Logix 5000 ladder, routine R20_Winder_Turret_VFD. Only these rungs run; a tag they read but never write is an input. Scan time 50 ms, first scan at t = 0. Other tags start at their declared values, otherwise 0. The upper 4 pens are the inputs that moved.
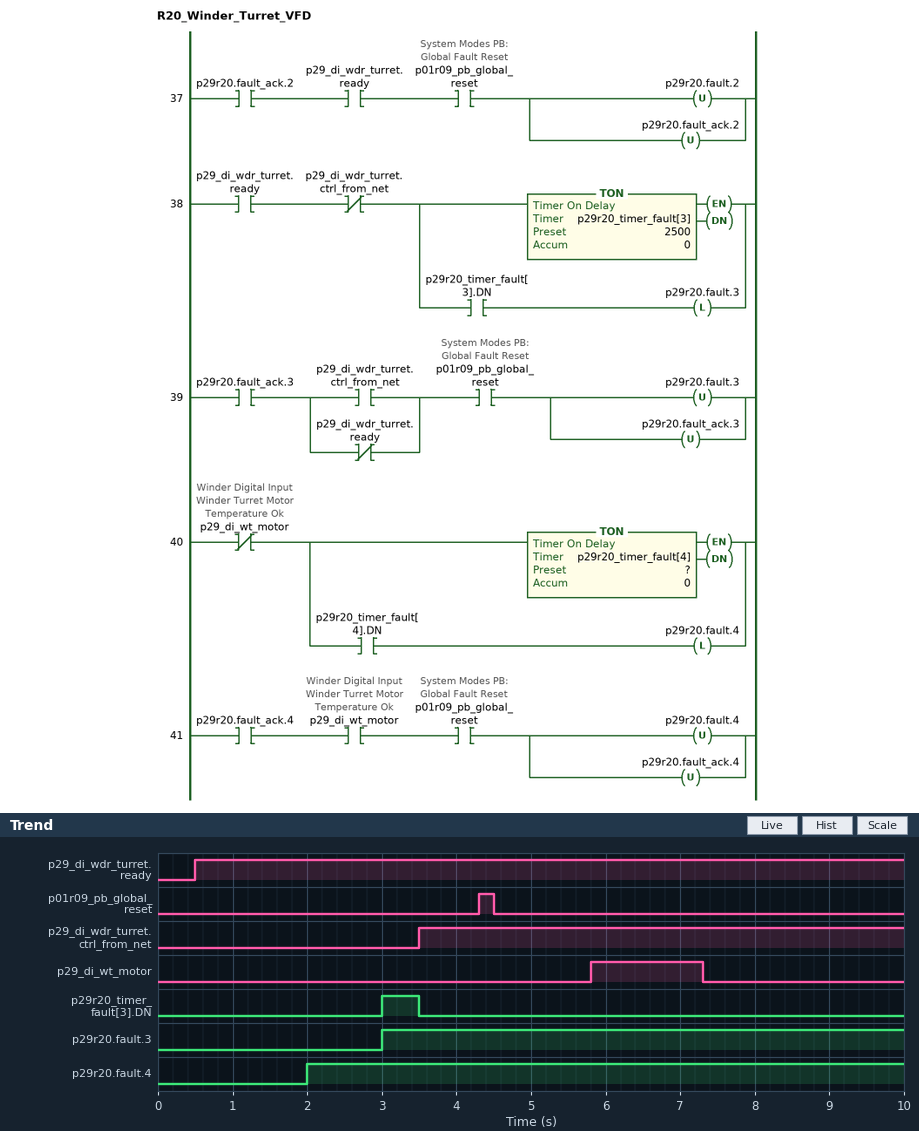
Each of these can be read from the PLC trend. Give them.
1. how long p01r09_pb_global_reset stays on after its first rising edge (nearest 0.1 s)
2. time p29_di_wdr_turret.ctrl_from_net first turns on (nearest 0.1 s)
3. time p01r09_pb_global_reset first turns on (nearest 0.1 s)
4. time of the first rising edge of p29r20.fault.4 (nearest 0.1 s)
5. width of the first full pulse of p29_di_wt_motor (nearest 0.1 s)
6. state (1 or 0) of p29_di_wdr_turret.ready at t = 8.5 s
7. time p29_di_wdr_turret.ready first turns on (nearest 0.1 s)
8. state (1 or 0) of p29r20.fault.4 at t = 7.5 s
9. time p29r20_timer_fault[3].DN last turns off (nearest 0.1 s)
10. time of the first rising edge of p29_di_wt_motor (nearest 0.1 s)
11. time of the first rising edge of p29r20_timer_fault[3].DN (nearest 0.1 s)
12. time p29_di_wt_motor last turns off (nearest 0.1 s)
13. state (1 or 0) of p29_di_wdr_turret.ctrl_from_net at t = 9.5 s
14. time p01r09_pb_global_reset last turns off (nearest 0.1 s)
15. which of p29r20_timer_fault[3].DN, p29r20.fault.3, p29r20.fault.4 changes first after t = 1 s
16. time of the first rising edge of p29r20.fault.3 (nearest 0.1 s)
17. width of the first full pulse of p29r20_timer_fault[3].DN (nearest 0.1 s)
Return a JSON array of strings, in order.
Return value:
["0.2 s", "3.5 s", "4.3 s", "2.0 s", "1.5 s", "1", "0.5 s", "1", "3.5 s", "5.8 s", "3.0 s", "7.3 s", "1", "4.5 s", "p29r20.fault.4", "3.0 s", "0.5 s"]
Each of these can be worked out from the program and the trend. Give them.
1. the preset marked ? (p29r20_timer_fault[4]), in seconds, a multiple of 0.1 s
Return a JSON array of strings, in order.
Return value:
["2.0 s"]
